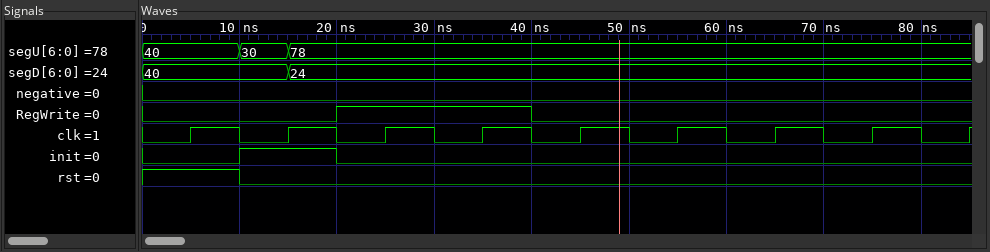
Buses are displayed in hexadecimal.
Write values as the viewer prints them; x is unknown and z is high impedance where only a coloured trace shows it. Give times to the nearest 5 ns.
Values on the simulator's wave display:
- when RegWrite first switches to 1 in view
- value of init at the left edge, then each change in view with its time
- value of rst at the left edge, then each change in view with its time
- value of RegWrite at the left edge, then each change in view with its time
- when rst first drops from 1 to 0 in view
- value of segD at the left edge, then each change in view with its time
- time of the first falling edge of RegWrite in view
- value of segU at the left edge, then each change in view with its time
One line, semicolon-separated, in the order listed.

20 ns; 0, 1 at 10 ns, 0 at 20 ns; 1, 0 at 10 ns; 0, 1 at 20 ns, 0 at 40 ns; 10 ns; 40, 24 at 15 ns; 40 ns; 40, 30 at 10 ns, 78 at 15 ns
